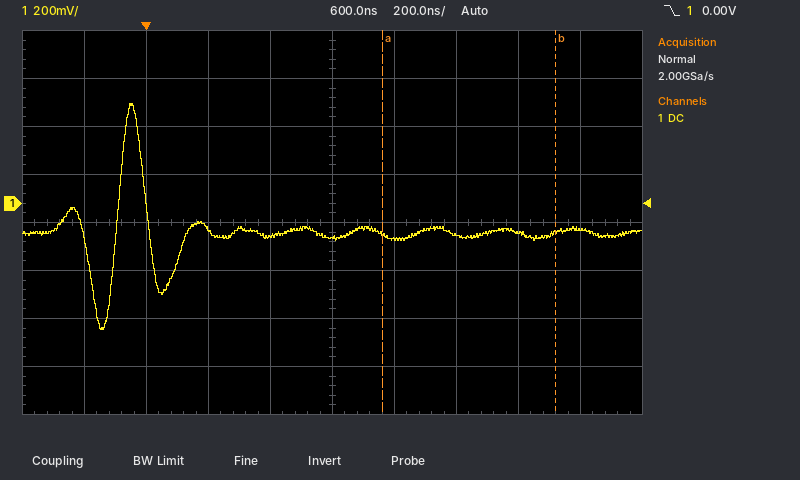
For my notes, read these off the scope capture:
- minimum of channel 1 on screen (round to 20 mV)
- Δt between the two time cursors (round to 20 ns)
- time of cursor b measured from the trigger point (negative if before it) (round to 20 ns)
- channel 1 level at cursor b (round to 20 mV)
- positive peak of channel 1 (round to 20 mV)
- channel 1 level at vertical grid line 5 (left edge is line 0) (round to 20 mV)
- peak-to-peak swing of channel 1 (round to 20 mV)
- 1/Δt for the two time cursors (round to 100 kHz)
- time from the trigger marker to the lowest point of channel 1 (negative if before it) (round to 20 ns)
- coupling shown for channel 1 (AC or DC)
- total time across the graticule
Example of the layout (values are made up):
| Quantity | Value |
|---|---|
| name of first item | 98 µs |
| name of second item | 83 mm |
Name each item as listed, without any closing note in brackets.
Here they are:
| Quantity | Value |
|---|---|
| minimum of channel 1 on screen | -520 mV |
| Δt between the two time cursors | 560 ns |
| time of cursor b measured from the trigger point (negative if before it) | +1.32 µs |
| channel 1 level at cursor b | -120 mV |
| positive peak of channel 1 | 420 mV |
| channel 1 level at vertical grid line 5 (left edge is line 0) | -140 mV |
| peak-to-peak swing of channel 1 | 940 mV |
| 1/Δt for the two time cursors | 1.8 MHz |
| time from the trigger marker to the lowest point of channel 1 (negative if before it) | -140 ns |
| coupling shown for channel 1 | DC |
| total time across the graticule | 2 µs |
